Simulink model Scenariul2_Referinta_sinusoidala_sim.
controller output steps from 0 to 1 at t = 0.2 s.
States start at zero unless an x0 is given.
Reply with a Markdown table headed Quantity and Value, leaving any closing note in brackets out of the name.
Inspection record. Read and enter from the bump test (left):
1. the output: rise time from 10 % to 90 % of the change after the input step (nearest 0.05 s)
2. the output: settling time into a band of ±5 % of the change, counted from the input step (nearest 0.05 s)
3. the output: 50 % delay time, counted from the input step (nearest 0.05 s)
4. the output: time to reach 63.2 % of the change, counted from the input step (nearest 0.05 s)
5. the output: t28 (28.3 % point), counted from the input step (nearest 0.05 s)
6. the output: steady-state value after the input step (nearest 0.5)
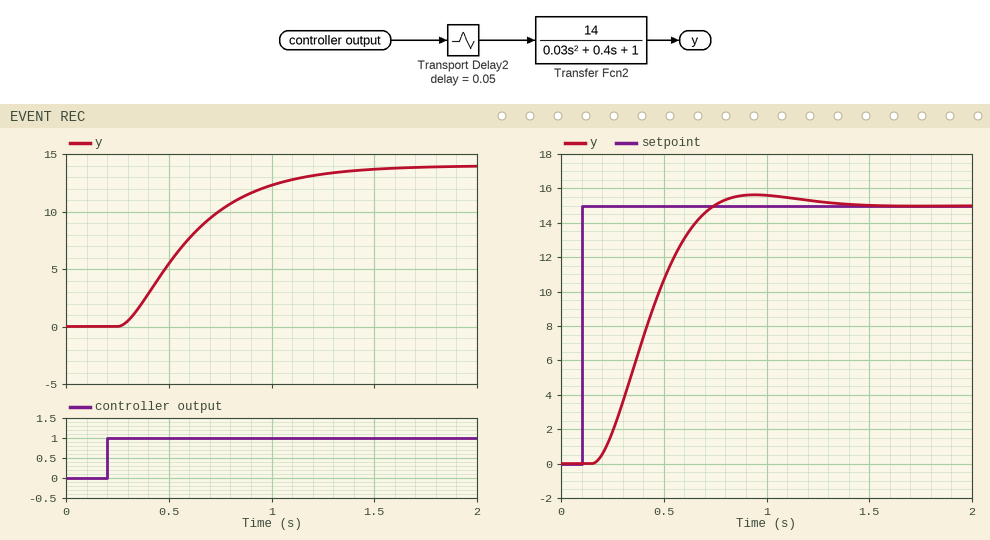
| Quantity | Value |
|---|---|
| the output: rise time from 10 % to 90 % of the change after the input step | 0.70 s |
| the output: settling time into a band of ±5 % of the change, counted from the input step | 1.05 s |
| the output: 50 % delay time, counted from the input step | 0.35 s |
| the output: time to reach 63.2 % of the change, counted from the input step | 0.45 s |
| the output: t28 (28.3 % point), counted from the input step | 0.25 s |
| the output: steady-state value after the input step | 14.0 |
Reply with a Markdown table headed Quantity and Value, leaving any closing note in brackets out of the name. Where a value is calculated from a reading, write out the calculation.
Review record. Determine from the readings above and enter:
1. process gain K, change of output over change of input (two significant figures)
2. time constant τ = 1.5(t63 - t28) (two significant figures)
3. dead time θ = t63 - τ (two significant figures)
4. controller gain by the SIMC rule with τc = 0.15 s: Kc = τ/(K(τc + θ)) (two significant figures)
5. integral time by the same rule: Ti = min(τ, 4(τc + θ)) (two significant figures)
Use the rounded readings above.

| Quantity | Value |
|---|---|
| process gain K, change of output over change of input | (14 - 0) / 1 = 14 |
| time constant τ = 1.5(t63 - t28) | 1.5 × (0.45 - 0.25) = 0.30 s |
| dead time θ = t63 - τ | 0.45 - 0.3 = 0.15 s |
| controller gain by the SIMC rule with τc = 0.15 s: Kc = τ/(K(τc + θ)) | 0.3 / (14 × (0.15 + 0.15)) = 0.071 |
| integral time by the same rule: Ti = min(τ, 4(τc + θ)) | min(0.3, 4 × (0.15 + 0.15)) = 0.30 s |
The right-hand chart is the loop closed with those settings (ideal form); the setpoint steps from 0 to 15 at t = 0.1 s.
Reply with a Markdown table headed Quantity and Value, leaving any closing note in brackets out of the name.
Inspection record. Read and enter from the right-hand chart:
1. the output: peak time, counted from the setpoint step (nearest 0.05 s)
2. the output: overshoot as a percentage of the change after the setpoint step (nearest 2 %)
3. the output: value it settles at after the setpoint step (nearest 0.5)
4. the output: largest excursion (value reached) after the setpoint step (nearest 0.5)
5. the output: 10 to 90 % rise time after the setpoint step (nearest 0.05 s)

| Quantity | Value |
|---|---|
| the output: peak time, counted from the setpoint step | 0.85 s |
| the output: overshoot as a percentage of the change after the setpoint step | 4 % |
| the output: value it settles at after the setpoint step | 15.0 |
| the output: largest excursion (value reached) after the setpoint step | 15.5 |
| the output: 10 to 90 % rise time after the setpoint step | 0.40 s |
